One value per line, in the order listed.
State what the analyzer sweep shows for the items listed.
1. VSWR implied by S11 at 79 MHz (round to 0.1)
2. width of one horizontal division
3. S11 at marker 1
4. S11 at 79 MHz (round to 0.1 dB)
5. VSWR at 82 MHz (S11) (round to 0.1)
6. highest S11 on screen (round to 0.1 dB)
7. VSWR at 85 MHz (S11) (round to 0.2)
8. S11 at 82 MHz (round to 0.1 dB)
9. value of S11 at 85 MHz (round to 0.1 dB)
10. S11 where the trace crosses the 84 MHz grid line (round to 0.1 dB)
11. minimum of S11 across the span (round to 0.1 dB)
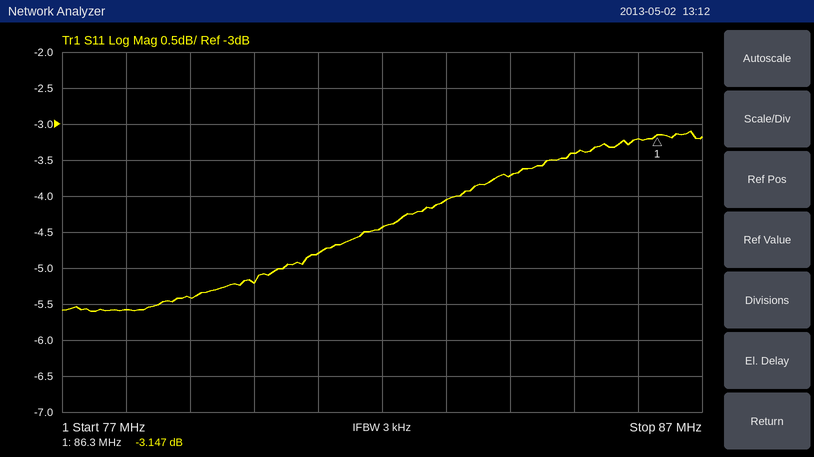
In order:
3.3
1 MHz
-3.147 dB
-5.4 dB
4.0
-3.1 dB
5.2
-4.4 dB
-3.4 dB
-3.7 dB
-5.6 dB
